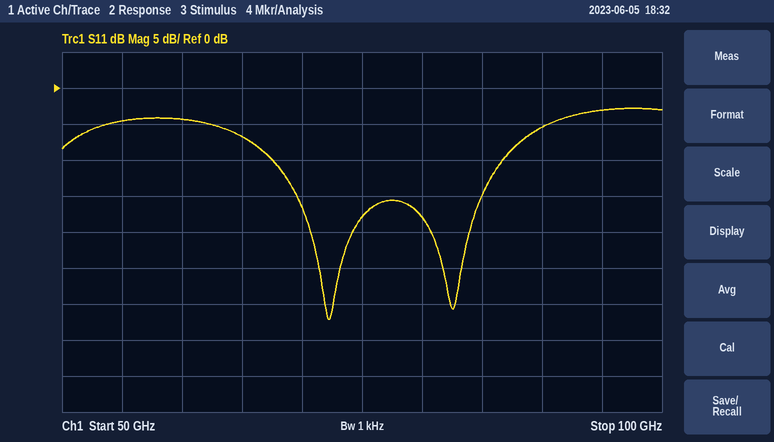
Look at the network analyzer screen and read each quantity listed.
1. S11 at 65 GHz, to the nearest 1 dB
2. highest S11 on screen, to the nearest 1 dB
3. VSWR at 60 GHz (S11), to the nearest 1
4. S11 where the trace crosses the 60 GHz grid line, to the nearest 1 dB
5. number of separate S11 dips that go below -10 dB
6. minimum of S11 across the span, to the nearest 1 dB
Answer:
-7 dB
-3 dB
4
-4 dB
2
-32 dB
